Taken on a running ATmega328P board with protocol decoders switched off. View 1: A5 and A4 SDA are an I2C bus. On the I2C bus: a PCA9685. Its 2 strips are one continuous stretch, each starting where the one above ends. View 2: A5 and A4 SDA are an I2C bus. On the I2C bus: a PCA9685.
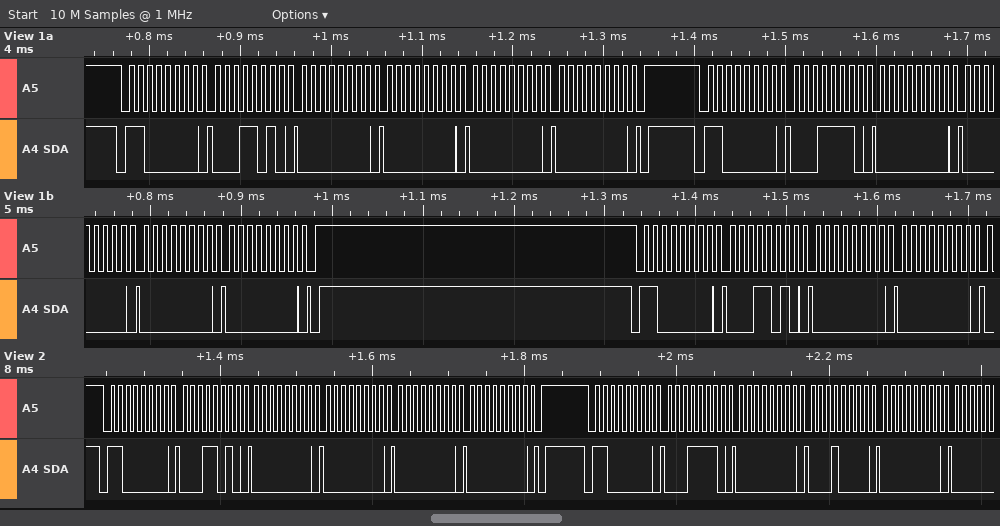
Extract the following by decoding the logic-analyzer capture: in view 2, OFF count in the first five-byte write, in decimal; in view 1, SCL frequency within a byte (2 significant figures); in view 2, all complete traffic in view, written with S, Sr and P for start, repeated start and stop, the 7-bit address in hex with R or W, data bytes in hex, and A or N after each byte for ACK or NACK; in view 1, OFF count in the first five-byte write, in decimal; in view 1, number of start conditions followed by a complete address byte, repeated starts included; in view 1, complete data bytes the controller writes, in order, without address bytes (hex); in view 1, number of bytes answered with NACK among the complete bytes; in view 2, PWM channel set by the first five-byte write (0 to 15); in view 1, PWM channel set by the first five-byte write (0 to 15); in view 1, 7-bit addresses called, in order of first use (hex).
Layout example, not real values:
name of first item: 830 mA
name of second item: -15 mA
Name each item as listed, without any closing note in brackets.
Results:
in view 2, OFF count in the first five-byte write, in decimal: 0
in view 1, SCL frequency within a byte: 100 kHz
in view 2, all complete traffic in view, written with S, Sr and P for start, repeated start and stop, the 7-bit address in hex with R or W, data bytes in hex, and A or N after each byte for ACK or NACK: S 60W A 1A A 00 A 00 A 00 A 00 A P S 60W A 1E A 00 A 10 A 00 A
in view 1, OFF count in the first five-byte write, in decimal: 0
in view 1, number of start conditions followed by a complete address byte, repeated starts included: 3
in view 1, complete data bytes the controller writes, in order, without address bytes: 1A 00 00 00 00 1E 00 00 00 00 1A 00 00
in view 1, number of bytes answered with NACK among the complete bytes: 0
in view 2, PWM channel set by the first five-byte write: 5
in view 1, PWM channel set by the first five-byte write: 5
in view 1, 7-bit addresses called, in order of first use: 0x60
